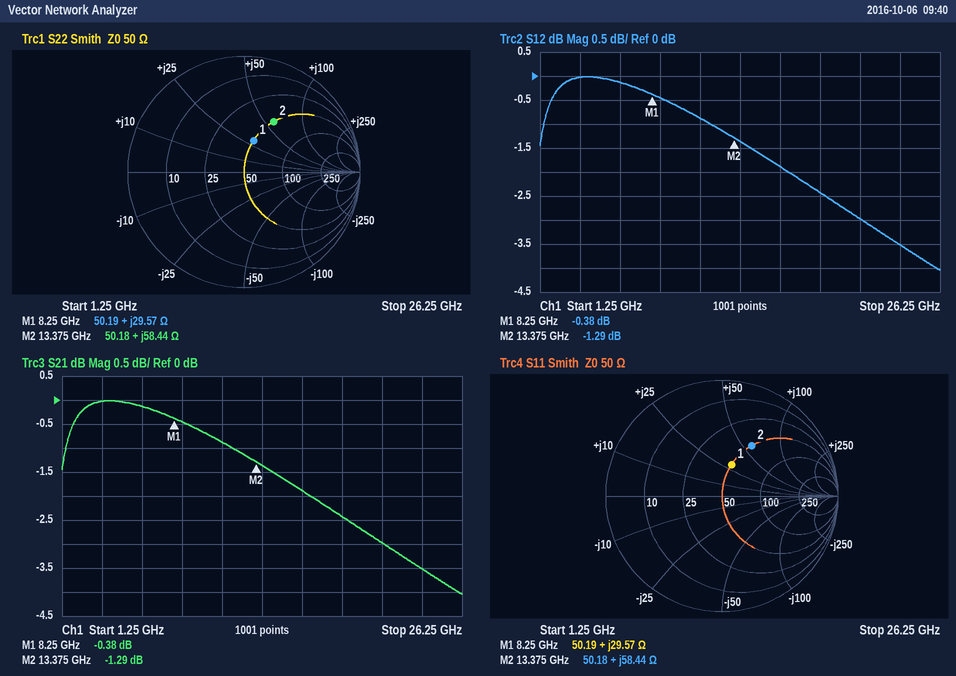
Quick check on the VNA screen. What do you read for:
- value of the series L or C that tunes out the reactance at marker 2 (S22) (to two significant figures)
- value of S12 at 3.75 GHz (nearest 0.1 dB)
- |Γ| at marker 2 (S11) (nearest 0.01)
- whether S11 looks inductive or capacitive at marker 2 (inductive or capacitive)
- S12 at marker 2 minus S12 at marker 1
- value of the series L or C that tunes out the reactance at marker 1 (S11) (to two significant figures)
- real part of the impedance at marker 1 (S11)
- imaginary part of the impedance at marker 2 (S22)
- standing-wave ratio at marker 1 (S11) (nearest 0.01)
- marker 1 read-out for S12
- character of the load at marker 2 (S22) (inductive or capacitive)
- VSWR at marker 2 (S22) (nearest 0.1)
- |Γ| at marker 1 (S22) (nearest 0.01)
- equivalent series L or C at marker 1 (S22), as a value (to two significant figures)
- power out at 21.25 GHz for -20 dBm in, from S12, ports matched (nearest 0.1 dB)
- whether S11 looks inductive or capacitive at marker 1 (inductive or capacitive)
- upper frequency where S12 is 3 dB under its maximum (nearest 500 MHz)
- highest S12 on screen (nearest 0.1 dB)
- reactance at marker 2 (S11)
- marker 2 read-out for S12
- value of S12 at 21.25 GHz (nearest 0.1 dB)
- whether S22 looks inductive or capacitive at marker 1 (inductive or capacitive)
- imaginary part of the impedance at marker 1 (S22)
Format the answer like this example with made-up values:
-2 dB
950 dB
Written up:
200 fF
0.0 dB
0.50
inductive
-0.91 dB
650 fF
50.19 Ω
+58.44 Ω
1.79
-0.38 dB
inductive
3.0
0.28
570 pH
-23.0 dBm
inductive
21.5 GHz
0.0 dB
+58.44 Ω
-1.29 dB
-3.0 dB
inductive
+29.57 Ω
